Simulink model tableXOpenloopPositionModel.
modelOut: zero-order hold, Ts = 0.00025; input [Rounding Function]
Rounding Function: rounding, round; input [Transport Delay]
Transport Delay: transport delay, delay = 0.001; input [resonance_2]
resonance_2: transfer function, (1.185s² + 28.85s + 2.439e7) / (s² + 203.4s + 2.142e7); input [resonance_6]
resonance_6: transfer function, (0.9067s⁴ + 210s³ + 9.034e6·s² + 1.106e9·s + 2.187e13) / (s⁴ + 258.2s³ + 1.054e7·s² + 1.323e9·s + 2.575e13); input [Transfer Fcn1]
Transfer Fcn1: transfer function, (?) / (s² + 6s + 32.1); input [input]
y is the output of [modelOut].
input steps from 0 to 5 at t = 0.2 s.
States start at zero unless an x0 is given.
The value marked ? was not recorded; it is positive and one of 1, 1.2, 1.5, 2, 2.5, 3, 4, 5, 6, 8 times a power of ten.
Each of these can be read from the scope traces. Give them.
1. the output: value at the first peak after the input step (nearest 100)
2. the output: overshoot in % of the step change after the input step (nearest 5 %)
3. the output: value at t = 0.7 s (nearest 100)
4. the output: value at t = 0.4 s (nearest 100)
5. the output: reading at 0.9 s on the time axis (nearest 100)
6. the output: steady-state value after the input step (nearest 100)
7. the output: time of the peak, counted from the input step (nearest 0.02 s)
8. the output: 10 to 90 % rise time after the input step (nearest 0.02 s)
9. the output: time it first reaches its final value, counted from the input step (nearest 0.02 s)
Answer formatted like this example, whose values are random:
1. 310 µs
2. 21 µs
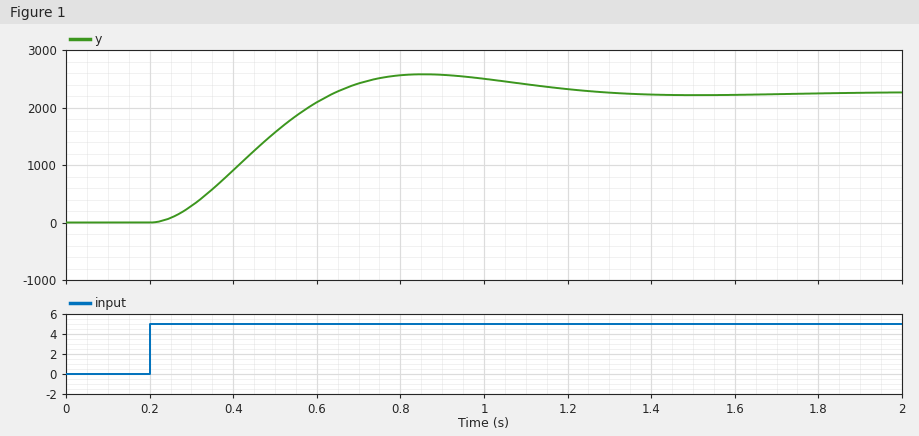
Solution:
1. 2600
2. 15 %
3. 2400
4. 900
5. 2600
6. 2300
7. 0.66 s
8. 0.30 s
9. 0.44 s
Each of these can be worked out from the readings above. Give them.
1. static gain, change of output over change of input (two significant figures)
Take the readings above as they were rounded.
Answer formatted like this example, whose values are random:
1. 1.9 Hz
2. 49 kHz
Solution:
1. 460
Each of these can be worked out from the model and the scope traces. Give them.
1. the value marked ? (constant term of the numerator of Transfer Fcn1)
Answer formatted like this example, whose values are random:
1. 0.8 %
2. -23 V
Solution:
1. 15000
